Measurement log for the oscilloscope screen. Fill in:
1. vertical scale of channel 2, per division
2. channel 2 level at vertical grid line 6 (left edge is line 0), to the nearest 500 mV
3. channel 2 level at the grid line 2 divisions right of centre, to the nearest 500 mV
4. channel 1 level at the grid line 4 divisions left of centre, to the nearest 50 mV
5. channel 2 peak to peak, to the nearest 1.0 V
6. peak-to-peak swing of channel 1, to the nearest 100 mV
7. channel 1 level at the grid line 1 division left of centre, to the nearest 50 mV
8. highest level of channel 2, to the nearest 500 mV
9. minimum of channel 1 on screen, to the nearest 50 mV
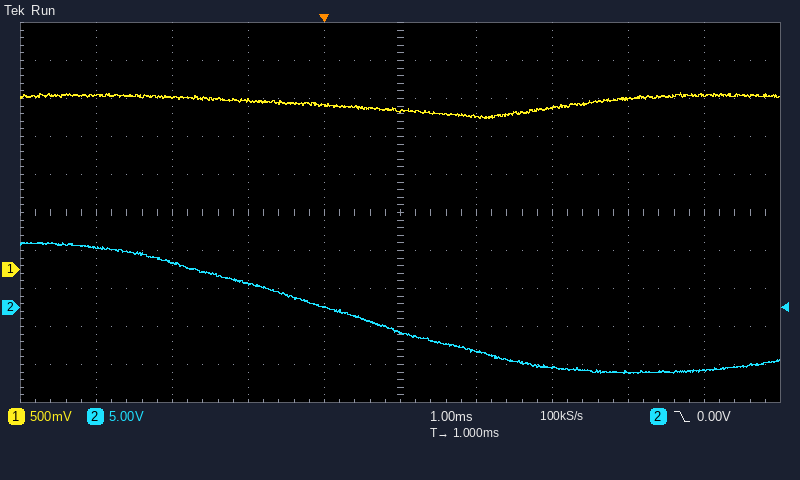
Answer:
5 V
-5.5 V
-8.0 V
2.30 V
17.0 V
300 mV
2.15 V
8.5 V
2.00 V
